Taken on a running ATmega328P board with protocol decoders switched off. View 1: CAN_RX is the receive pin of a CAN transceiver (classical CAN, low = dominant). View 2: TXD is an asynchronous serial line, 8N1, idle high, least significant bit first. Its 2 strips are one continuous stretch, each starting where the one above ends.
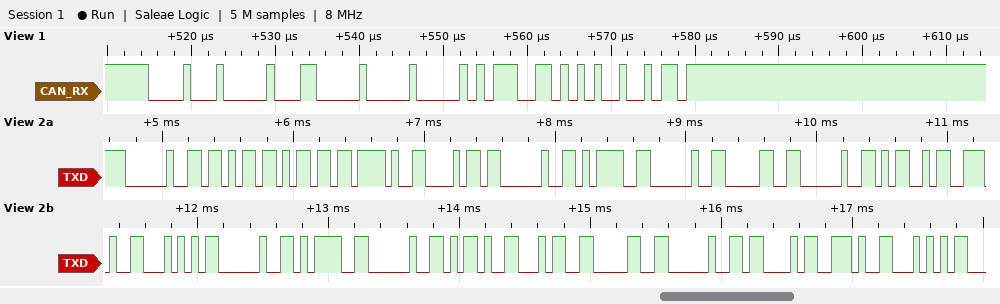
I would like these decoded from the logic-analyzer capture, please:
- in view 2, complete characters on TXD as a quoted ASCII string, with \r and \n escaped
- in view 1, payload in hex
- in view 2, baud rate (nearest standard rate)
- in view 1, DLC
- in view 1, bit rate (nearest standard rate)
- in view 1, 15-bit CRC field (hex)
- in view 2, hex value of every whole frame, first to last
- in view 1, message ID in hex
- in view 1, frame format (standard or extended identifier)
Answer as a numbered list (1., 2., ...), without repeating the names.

1. " km/h = 0 M.T = -40 C.T"
2. 00 00 B9
3. 19200 baud
4. 3
5. 1000 kbit/s
6. 0x5525
7. 20 6B 6D 2F 68 20 3D 20 30 20 4D 2E 54 20 3D 20 2D 34 30 20 43 2E 54
8. 0x088
9. standard
